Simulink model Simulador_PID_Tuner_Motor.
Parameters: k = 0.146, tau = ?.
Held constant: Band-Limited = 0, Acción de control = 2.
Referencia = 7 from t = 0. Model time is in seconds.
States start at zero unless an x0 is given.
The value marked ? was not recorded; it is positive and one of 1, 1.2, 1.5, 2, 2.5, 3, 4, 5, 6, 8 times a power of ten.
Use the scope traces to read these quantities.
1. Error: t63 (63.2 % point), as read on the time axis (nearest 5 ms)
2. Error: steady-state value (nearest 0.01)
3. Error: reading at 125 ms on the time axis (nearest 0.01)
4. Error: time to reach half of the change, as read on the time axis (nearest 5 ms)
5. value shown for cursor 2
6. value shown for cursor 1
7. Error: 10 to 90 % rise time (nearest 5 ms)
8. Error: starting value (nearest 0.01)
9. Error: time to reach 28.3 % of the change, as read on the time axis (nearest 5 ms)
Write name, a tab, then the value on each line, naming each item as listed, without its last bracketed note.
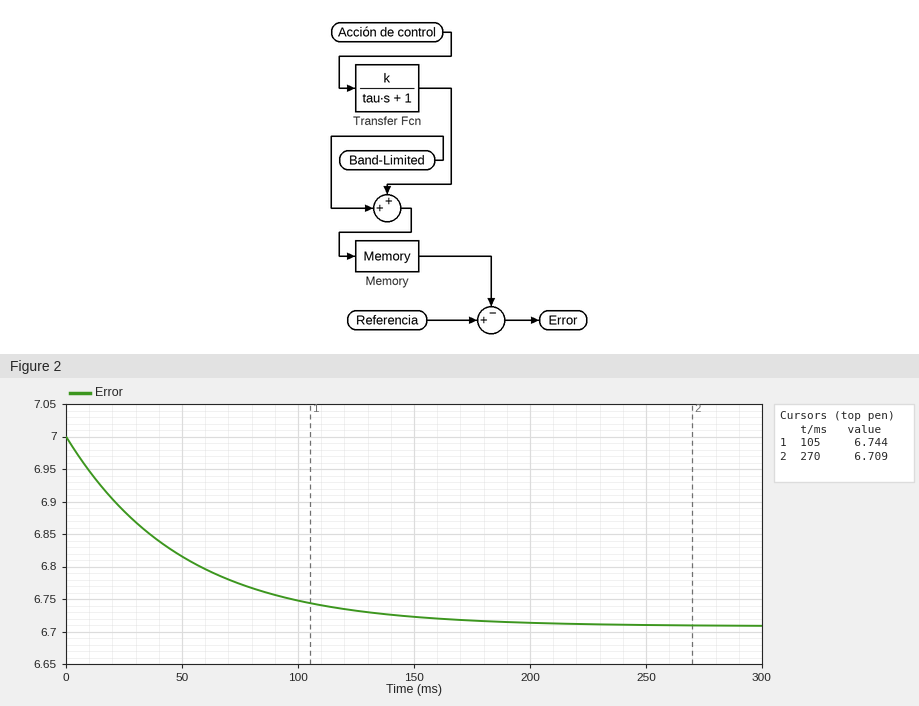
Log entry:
Error: t63 (63.2 % point), as read on the time axis	50 ms
Error: steady-state value	6.71
Error: reading at 125 ms on the time axis	6.73
Error: time to reach half of the change, as read on the time axis	35 ms
value shown for cursor 2	6.709
value shown for cursor 1	6.744
Error: 10 to 90 % rise time	110 ms
Error: starting value	7.00
Error: time to reach 28.3 % of the change, as read on the time axis	15 ms
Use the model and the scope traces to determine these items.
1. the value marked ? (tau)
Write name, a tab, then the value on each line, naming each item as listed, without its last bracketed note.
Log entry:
the value marked ?	0.05
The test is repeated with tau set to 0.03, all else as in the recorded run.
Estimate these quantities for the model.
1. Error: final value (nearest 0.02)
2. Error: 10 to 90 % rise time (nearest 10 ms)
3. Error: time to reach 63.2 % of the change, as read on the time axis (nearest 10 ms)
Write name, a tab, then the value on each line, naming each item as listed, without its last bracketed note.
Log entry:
Error: final value	6.70
Error: 10 to 90 % rise time	70 ms
Error: time to reach 63.2 % of the change, as read on the time axis	30 ms
